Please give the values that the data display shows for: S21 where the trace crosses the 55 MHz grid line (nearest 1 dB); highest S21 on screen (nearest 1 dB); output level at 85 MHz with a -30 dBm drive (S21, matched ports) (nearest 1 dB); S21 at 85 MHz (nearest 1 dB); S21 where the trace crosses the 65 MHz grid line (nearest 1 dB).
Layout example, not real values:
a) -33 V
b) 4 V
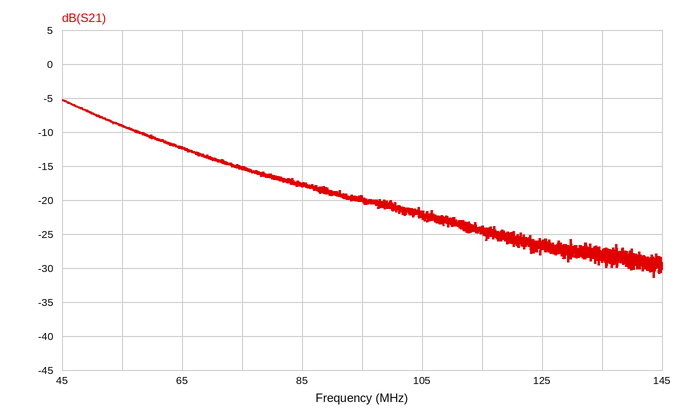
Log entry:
a) -9 dB
b) -5 dB
c) -48 dBm
d) -18 dB
e) -12 dB
